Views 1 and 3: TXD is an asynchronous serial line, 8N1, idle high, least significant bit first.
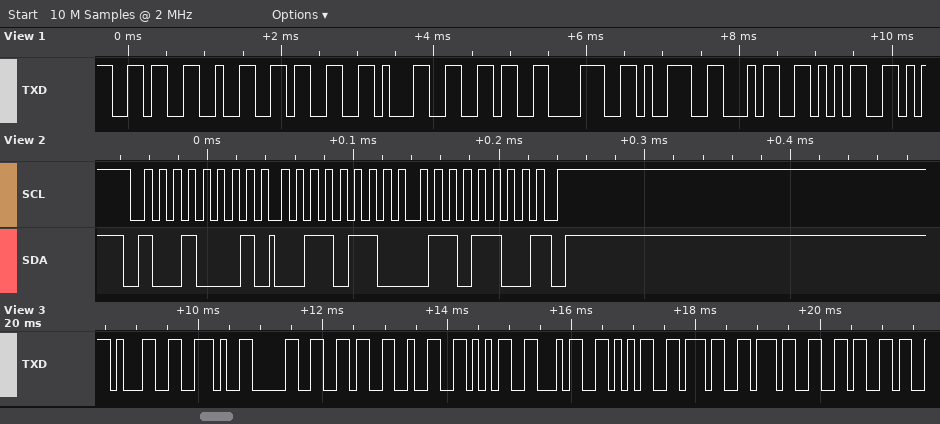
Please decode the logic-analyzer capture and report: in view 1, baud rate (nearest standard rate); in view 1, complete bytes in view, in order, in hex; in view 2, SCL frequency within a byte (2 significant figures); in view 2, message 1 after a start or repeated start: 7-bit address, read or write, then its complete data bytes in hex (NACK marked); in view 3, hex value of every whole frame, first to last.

9600 baud
36 32 33 31 36 38 39 34 35
100 kHz
0x48 read: 36 6C NACK
31 2E 30 36 32 35 34 35 37 37 36
